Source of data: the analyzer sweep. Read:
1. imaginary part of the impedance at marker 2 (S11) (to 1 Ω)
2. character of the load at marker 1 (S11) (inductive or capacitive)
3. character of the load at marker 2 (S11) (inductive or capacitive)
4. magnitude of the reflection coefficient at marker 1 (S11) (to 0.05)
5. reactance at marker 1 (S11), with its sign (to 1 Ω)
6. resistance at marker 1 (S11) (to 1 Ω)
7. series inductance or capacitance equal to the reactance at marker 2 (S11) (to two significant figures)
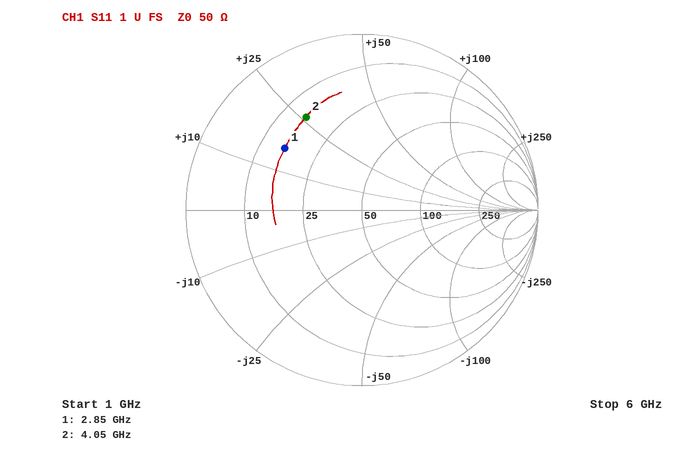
+26 Ω
inductive
inductive
0.55
+16 Ω
16 Ω
1.0 nH
